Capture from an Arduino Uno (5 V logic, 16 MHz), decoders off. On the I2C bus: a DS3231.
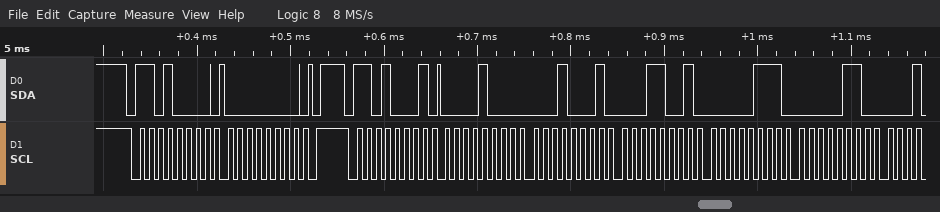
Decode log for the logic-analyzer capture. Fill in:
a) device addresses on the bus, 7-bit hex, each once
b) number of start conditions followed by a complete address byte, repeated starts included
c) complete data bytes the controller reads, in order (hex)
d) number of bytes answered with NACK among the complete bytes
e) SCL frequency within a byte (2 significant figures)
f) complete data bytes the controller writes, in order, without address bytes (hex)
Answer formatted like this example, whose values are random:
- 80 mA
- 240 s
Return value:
- 0x68
- 2
- 08 11 19 07 06
- 0
- 100 kHz
- 00
